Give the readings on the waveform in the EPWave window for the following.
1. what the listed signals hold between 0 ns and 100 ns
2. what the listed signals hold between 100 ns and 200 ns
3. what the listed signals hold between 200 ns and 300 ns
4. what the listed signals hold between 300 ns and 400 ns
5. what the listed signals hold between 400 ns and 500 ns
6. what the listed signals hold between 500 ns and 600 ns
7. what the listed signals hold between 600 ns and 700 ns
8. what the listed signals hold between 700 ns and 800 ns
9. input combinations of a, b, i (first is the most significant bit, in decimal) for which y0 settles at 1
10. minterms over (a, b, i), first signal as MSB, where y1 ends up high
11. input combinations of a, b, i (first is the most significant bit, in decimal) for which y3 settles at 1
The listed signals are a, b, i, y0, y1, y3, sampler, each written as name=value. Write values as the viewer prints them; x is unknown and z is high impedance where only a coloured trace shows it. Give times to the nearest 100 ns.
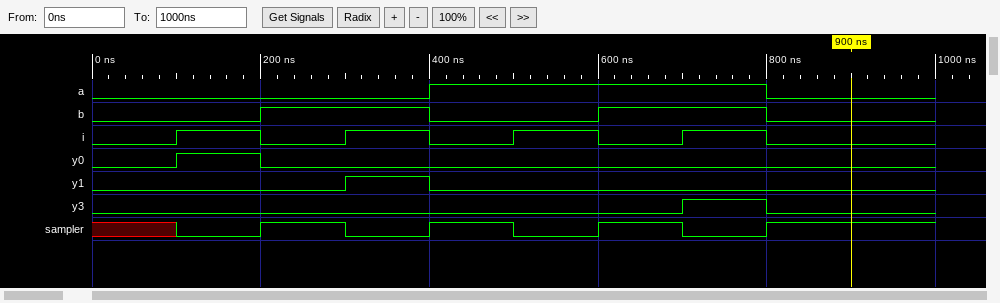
a=0, b=0, i=0, y0=0, y1=0, y3=0, sampler=x
a=0, b=0, i=1, y0=1, y1=0, y3=0, sampler=0
a=0, b=1, i=0, y0=0, y1=0, y3=0, sampler=1
a=0, b=1, i=1, y0=0, y1=1, y3=0, sampler=0
a=1, b=0, i=0, y0=0, y1=0, y3=0, sampler=1
a=1, b=0, i=1, y0=0, y1=0, y3=0, sampler=0
a=1, b=1, i=0, y0=0, y1=0, y3=0, sampler=1
a=1, b=1, i=1, y0=0, y1=0, y3=1, sampler=0
1
3
7
